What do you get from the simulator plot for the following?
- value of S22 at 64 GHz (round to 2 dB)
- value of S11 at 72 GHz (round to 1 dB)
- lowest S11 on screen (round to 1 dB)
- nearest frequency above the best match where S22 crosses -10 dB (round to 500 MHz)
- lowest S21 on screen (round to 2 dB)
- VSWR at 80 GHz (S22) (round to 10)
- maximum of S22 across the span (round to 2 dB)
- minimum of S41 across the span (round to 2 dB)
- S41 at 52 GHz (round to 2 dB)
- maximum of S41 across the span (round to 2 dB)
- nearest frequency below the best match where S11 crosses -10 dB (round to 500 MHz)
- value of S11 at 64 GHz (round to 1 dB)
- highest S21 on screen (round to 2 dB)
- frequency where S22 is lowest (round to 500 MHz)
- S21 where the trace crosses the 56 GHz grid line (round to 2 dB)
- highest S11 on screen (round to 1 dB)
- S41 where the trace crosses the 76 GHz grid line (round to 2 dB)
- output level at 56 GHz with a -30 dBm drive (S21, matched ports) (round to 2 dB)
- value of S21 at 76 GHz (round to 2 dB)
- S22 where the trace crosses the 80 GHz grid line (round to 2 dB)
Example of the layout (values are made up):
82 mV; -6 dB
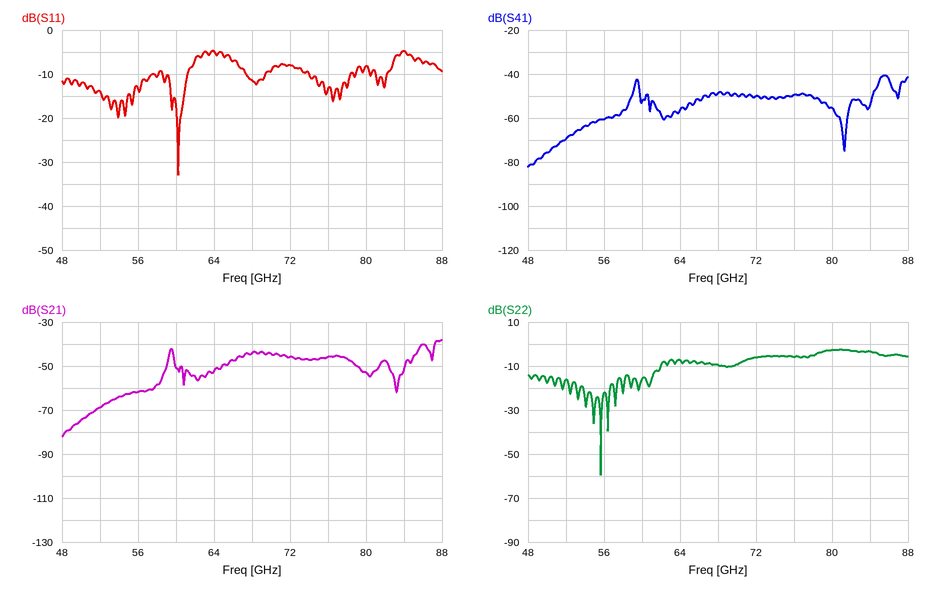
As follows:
-8 dB; -8 dB; -33 dB; 62.0 GHz; -82 dB; 10; -2 dB; -82 dB; -70 dB; -40 dB; 58.5 GHz; -5 dB; -38 dB; 55.5 GHz; -62 dB; -5 dB; -50 dB; -92 dBm; -46 dB; -2 dB
